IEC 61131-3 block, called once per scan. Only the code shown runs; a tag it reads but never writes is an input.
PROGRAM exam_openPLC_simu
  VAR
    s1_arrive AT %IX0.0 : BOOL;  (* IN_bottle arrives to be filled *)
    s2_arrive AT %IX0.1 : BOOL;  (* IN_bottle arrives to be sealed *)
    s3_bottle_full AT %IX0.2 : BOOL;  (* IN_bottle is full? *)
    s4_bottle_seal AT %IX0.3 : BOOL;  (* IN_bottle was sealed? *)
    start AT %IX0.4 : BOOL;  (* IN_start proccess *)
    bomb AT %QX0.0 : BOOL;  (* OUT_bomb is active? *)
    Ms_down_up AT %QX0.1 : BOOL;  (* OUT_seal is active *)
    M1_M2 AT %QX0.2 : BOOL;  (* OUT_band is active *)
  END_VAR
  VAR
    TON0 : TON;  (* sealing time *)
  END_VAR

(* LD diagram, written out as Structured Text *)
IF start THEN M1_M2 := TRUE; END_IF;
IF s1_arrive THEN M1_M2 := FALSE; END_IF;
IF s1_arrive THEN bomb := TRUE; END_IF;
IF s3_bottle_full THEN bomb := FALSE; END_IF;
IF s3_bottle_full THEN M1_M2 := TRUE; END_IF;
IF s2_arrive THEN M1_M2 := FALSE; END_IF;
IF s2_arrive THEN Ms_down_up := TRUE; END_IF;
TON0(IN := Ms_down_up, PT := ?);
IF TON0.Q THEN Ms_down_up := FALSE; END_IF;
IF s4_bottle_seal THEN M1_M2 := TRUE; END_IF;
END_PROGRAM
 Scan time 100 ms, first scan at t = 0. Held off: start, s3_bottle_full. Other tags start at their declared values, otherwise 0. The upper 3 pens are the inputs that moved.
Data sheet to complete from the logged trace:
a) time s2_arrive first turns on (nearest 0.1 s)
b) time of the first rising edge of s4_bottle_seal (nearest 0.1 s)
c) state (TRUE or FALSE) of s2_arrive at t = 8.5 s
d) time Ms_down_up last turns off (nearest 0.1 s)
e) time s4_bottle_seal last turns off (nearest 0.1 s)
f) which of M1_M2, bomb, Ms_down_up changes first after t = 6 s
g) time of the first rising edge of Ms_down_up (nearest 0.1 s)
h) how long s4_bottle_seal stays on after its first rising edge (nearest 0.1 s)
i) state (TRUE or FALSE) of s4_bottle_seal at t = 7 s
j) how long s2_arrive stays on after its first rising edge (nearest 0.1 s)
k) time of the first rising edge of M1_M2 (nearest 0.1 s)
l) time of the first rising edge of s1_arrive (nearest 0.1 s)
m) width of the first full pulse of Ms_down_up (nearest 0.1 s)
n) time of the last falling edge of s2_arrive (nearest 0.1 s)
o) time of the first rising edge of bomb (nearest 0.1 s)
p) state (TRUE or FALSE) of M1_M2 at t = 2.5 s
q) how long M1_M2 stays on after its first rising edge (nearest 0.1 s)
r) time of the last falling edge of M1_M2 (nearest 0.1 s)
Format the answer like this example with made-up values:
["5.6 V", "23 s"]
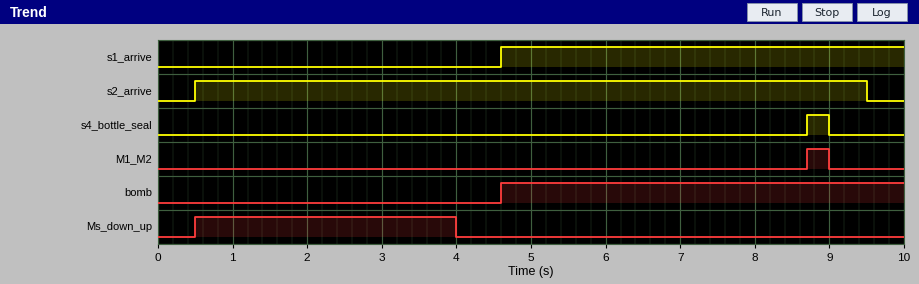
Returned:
["0.5 s", "8.7 s", "TRUE", "4.0 s", "9.0 s", "M1_M2", "0.5 s", "0.3 s", "FALSE", "9.0 s", "8.7 s", "4.6 s", "3.5 s", "9.5 s", "4.6 s", "FALSE", "0.3 s", "9.0 s"]
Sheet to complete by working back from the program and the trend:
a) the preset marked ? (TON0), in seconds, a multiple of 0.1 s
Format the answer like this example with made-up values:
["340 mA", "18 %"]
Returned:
["3.5 s"]
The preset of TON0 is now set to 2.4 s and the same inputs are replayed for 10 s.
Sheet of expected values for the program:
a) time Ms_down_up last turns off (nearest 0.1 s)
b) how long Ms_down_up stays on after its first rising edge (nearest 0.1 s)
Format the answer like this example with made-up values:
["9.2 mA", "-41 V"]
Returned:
["2.9 s", "2.4 s"]
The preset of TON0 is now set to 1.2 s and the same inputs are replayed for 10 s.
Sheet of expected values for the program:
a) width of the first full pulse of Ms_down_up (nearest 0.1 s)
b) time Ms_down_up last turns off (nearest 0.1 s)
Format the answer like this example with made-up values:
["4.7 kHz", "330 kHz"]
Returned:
["1.2 s", "1.7 s"]
